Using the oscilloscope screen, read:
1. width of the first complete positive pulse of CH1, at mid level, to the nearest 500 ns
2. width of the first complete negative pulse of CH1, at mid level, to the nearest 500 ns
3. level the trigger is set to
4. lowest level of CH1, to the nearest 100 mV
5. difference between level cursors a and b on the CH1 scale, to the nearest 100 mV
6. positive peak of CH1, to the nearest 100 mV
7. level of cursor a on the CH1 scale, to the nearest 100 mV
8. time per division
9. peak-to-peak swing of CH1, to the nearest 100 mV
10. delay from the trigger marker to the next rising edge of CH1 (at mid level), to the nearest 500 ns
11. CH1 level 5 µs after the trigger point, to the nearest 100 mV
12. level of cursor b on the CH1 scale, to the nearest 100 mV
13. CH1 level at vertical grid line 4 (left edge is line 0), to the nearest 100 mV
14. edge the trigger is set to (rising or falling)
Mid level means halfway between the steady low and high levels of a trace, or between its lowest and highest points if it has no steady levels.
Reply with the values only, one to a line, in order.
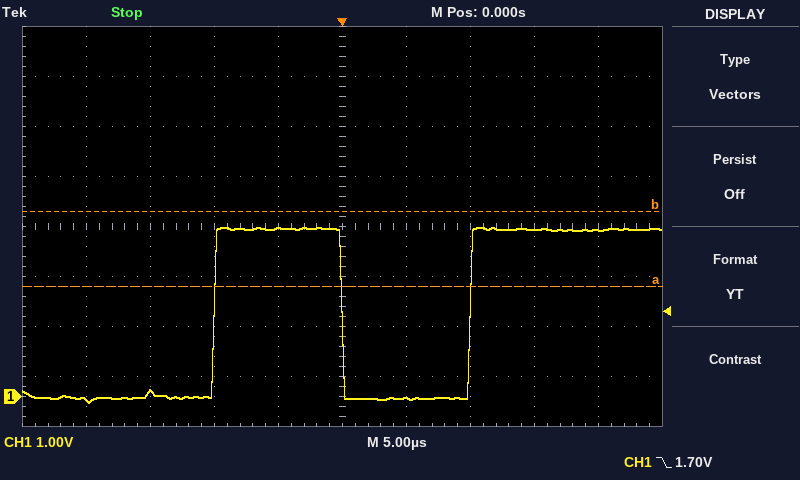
10.0 µs
10.0 µs
1.70 V
-100 mV
1.5 V
3.4 V
2.2 V
5 µs
3.5 V
10.0 µs
0.0 V
3.7 V
3.4 V
falling
